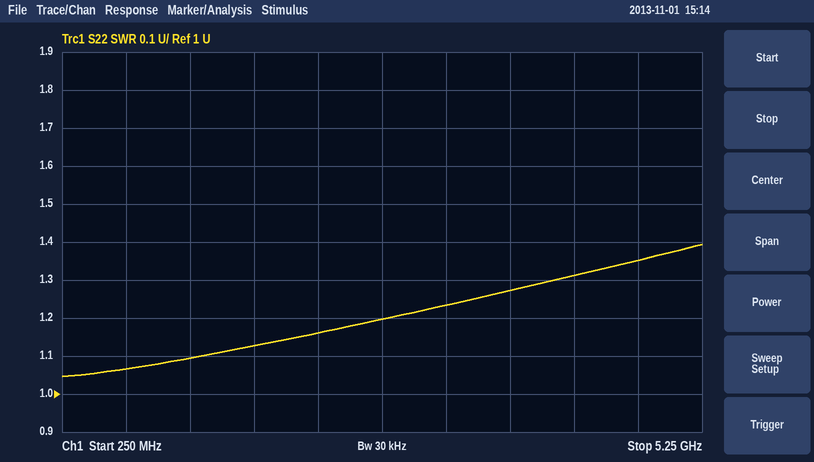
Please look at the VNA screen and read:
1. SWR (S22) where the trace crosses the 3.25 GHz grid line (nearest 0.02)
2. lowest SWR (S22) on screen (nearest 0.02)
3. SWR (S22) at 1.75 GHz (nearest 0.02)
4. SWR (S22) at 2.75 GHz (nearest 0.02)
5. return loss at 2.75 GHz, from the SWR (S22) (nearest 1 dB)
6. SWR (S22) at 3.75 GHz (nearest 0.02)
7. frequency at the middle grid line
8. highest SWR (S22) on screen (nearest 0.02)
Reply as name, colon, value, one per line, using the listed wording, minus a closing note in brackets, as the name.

SWR (S22) where the trace crosses the 3.25 GHz grid line: 1.24
lowest SWR (S22) on screen: 1.04
SWR (S22) at 1.75 GHz: 1.12
SWR (S22) at 2.75 GHz: 1.20
return loss at 2.75 GHz, from the SWR (S22): 21 dB
SWR (S22) at 3.75 GHz: 1.28
frequency at the middle grid line: 2.75 GHz
highest SWR (S22) on screen: 1.40
